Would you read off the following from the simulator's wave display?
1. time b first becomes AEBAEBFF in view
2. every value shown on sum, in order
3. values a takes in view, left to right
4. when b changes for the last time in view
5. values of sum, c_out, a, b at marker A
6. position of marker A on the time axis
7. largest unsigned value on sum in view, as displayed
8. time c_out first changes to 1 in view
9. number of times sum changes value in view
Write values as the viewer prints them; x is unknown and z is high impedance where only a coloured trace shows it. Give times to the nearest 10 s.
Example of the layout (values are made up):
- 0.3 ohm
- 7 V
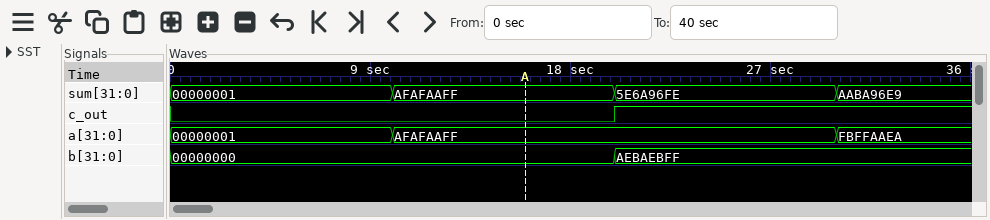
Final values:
- 20 s
- 00000001, AFAFAAFF, 5E6A96FE, AABA96E9
- 00000001, AFAFAAFF, FBFFAAEA
- 20 s
- sum=AFAFAAFF, c_out=0, a=AFAFAAFF, b=00000000
- 20 s
- AFAFAAFF
- 20 s
- 3
